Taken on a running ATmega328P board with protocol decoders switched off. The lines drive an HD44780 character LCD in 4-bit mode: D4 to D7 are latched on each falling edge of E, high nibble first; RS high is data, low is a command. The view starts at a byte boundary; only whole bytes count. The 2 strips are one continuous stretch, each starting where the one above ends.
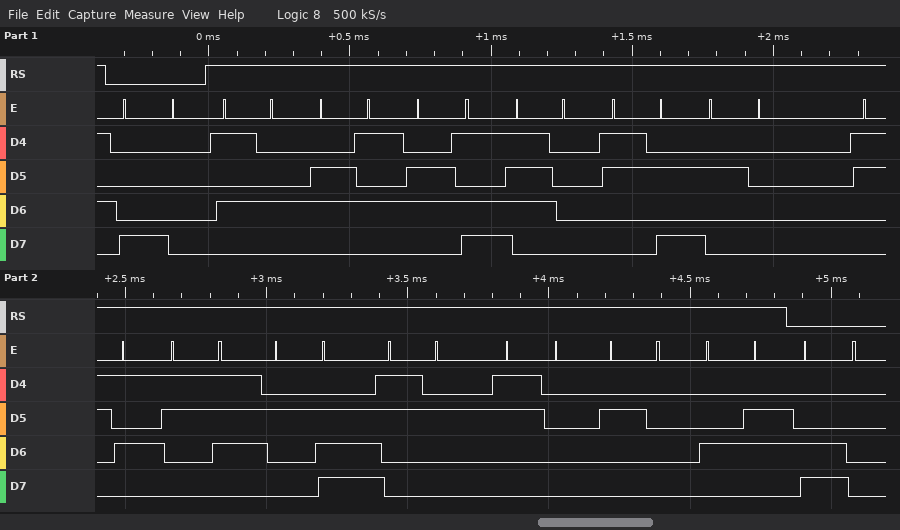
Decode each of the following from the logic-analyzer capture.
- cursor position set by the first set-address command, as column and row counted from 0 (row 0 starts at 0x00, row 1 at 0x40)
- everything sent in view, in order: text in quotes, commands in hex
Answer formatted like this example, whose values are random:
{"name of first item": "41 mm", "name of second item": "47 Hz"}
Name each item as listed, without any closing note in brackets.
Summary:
{"cursor position set by the first set-address command, as column and row counted from 0": "column 0, row 0", "everything sent in view, in order: text in quotes, commands in hex": "0x80 \"Temp: 57.20 F\" 0xC0"}
